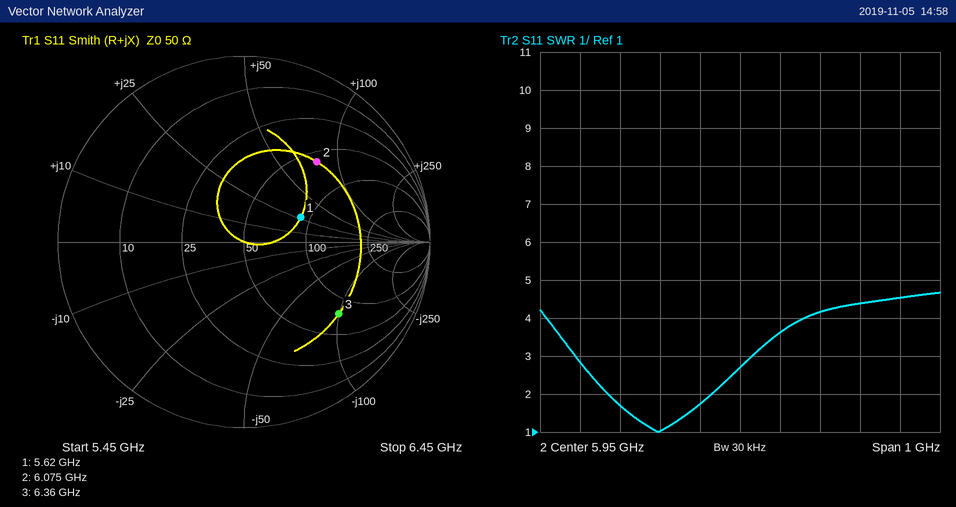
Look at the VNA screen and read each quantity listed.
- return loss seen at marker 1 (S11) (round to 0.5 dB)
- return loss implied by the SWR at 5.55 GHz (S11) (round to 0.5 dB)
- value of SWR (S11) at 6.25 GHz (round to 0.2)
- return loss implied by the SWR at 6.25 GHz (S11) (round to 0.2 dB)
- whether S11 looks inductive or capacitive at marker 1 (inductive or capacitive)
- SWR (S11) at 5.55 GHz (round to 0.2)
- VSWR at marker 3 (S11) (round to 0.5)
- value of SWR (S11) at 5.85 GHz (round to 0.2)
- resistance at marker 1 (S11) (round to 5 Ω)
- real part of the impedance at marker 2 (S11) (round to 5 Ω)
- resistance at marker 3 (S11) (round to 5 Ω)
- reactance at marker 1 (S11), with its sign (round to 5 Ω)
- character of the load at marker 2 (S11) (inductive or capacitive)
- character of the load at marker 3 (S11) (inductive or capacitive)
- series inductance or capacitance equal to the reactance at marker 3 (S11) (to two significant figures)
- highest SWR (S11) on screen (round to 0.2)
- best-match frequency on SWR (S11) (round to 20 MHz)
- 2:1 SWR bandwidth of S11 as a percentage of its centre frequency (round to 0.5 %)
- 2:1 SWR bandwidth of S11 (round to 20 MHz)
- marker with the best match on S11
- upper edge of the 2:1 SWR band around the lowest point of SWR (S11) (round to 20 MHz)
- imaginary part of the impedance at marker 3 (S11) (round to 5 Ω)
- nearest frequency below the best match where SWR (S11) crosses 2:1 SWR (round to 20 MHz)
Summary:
9.5 dB
6.5 dB
4.4
4.0 dB
inductive
2.8
4.5
1.8
90 Ω
60 Ω
75 Ω
+25 Ω
inductive
capacitive
250 fF
4.6
5.74 GHz
4.5 %
260 MHz
marker 1
5.88 GHz
-100 Ω
5.62 GHz
